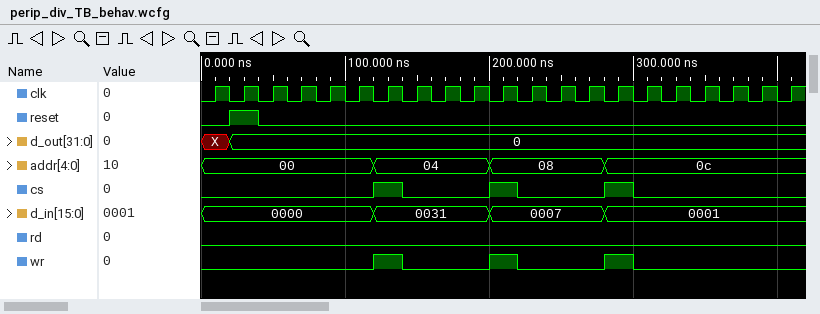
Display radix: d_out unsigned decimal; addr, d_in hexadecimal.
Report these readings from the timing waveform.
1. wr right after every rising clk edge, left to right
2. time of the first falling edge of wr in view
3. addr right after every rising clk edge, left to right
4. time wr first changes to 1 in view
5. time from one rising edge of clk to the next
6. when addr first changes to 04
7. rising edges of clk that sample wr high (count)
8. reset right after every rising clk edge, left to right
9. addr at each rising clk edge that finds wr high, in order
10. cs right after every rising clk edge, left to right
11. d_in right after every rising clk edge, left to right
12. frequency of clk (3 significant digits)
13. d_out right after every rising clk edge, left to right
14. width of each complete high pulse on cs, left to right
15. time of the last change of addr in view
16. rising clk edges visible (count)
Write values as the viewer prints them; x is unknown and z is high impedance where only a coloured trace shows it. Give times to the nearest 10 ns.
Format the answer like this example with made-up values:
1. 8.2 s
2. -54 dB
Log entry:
1. 0 0 0 0 0 0 1 0 0 0 1 0 0 0 1 0 0 0 0 0 0
2. 140 ns
3. 00, 00, 00, 00, 00, 00, 04, 04, 04, 04, 08, 08, 08, 08, 0c, 0c, 0c, 0c, 0c, 0c, 0c
4. 120 ns
5. 20 ns
6. 120 ns
7. 3
8. 0 1 0 0 0 0 0 0 0 0 0 0 0 0 0 0 0 0 0 0 0
9. 04, 08, 0c
10. 0 0 0 0 0 0 1 0 0 0 1 0 0 0 1 0 0 0 0 0 0
11. 0000, 0000, 0000, 0000, 0000, 0000, 0031, 0031, 0031, 0031, 0007, 0007, 0007, 0007, 0001, 0001, 0001, 0001, 0001, 0001, 0001
12. 50.0 MHz
13. X, 0, 0, 0, 0, 0, 0, 0, 0, 0, 0, 0, 0, 0, 0, 0, 0, 0, 0, 0, 0
14. 20 ns, 20 ns, 20 ns
15. 280 ns
16. 21
